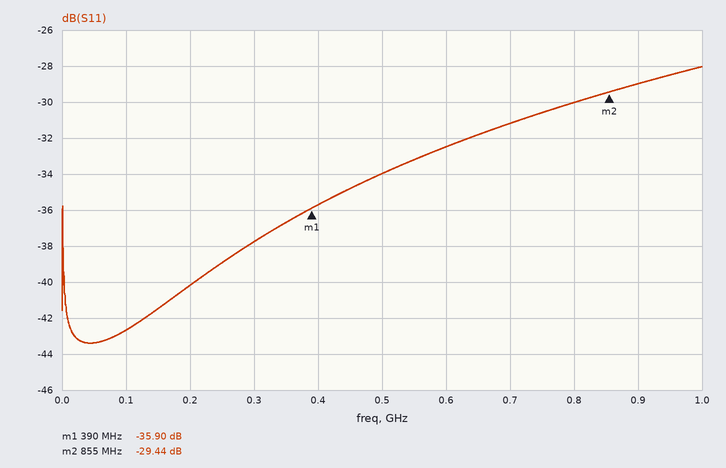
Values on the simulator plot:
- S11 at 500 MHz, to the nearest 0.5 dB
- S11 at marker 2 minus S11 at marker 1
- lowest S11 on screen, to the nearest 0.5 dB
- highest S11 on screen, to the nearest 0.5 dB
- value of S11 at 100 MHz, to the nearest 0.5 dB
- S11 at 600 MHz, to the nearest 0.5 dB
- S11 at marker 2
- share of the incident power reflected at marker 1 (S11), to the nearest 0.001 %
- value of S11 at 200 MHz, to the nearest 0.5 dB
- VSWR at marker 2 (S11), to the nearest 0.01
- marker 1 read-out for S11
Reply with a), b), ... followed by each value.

a) -34.0 dB
b) 6.46 dB
c) -43.5 dB
d) -28.0 dB
e) -42.5 dB
f) -32.5 dB
g) -29.44 dB
h) 0.026 %
i) -40.0 dB
j) 1.07
k) -35.90 dB
